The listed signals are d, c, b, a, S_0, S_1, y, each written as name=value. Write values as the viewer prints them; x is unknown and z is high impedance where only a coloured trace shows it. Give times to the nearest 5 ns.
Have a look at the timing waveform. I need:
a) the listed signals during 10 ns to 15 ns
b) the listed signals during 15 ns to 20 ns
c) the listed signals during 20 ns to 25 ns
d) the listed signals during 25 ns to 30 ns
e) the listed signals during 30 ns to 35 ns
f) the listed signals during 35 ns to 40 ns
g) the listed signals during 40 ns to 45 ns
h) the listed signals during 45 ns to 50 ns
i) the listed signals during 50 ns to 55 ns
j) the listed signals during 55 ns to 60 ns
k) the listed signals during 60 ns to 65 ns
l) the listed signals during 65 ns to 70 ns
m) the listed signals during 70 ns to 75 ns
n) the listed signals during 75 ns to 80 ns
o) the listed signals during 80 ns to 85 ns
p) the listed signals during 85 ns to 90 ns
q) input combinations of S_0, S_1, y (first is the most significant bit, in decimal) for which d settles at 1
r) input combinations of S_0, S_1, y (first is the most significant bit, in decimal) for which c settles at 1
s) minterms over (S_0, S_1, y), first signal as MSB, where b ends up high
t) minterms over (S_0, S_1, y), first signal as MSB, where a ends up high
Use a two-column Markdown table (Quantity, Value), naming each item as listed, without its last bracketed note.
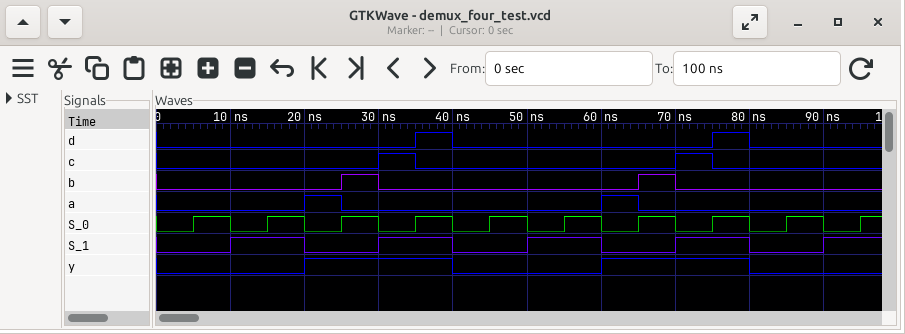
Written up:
| Quantity | Value |
|---|---|
| the listed signals during 10 ns to 15 ns | d=0, c=0, b=0, a=0, S_0=0, S_1=1, y=0 |
| the listed signals during 15 ns to 20 ns | d=0, c=0, b=0, a=0, S_0=1, S_1=1, y=0 |
| the listed signals during 20 ns to 25 ns | d=0, c=0, b=0, a=1, S_0=0, S_1=0, y=1 |
| the listed signals during 25 ns to 30 ns | d=0, c=0, b=1, a=0, S_0=1, S_1=0, y=1 |
| the listed signals during 30 ns to 35 ns | d=0, c=1, b=0, a=0, S_0=0, S_1=1, y=1 |
| the listed signals during 35 ns to 40 ns | d=1, c=0, b=0, a=0, S_0=1, S_1=1, y=1 |
| the listed signals during 40 ns to 45 ns | d=0, c=0, b=0, a=0, S_0=0, S_1=0, y=0 |
| the listed signals during 45 ns to 50 ns | d=0, c=0, b=0, a=0, S_0=1, S_1=0, y=0 |
| the listed signals during 50 ns to 55 ns | d=0, c=0, b=0, a=0, S_0=0, S_1=1, y=0 |
| the listed signals during 55 ns to 60 ns | d=0, c=0, b=0, a=0, S_0=1, S_1=1, y=0 |
| the listed signals during 60 ns to 65 ns | d=0, c=0, b=0, a=1, S_0=0, S_1=0, y=1 |
| the listed signals during 65 ns to 70 ns | d=0, c=0, b=1, a=0, S_0=1, S_1=0, y=1 |
| the listed signals during 70 ns to 75 ns | d=0, c=1, b=0, a=0, S_0=0, S_1=1, y=1 |
| the listed signals during 75 ns to 80 ns | d=1, c=0, b=0, a=0, S_0=1, S_1=1, y=1 |
| the listed signals during 80 ns to 85 ns | d=0, c=0, b=0, a=0, S_0=0, S_1=0, y=0 |
| the listed signals during 85 ns to 90 ns | d=0, c=0, b=0, a=0, S_0=1, S_1=0, y=0 |
| input combinations of S_0, S_1, y (first is the most significant bit, in decimal) for which d settles at 1 | 7 |
| input combinations of S_0, S_1, y (first is the most significant bit, in decimal) for which c settles at 1 | 3 |
| minterms over (S_0, S_1, y), first signal as MSB, where b ends up high | 5 |
| minterms over (S_0, S_1, y), first signal as MSB, where a ends up high | 1 |
